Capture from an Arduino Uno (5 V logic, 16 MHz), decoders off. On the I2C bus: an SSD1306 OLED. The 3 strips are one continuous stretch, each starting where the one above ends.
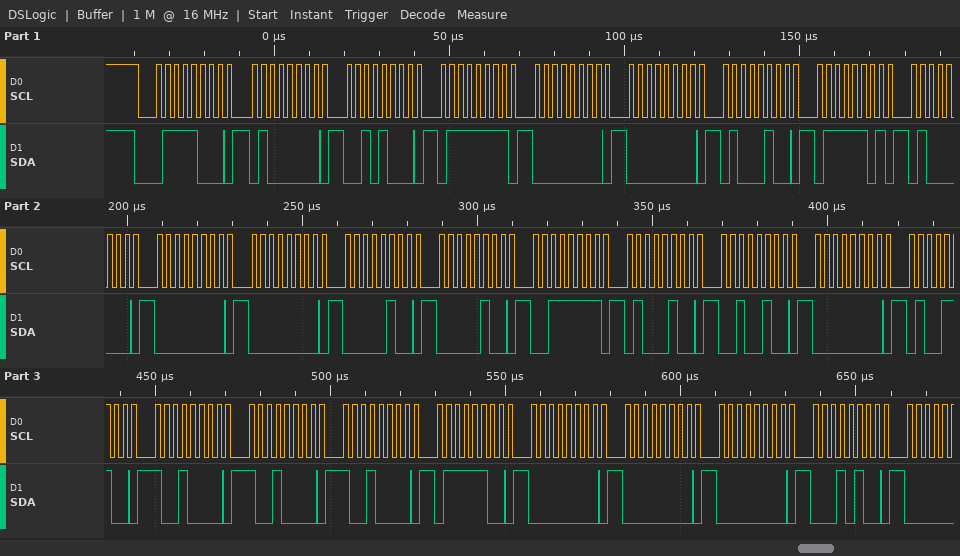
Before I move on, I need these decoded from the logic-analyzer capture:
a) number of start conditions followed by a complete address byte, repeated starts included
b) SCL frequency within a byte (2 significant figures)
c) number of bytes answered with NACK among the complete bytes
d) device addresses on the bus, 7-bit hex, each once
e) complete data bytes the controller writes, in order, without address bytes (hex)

1
400 kHz
0
0x3C
40 28 7F 00 00 44 7D 40 00 00 04 04 3F 44 24 00 4C 90 90 90 7C 00 00 00 14
